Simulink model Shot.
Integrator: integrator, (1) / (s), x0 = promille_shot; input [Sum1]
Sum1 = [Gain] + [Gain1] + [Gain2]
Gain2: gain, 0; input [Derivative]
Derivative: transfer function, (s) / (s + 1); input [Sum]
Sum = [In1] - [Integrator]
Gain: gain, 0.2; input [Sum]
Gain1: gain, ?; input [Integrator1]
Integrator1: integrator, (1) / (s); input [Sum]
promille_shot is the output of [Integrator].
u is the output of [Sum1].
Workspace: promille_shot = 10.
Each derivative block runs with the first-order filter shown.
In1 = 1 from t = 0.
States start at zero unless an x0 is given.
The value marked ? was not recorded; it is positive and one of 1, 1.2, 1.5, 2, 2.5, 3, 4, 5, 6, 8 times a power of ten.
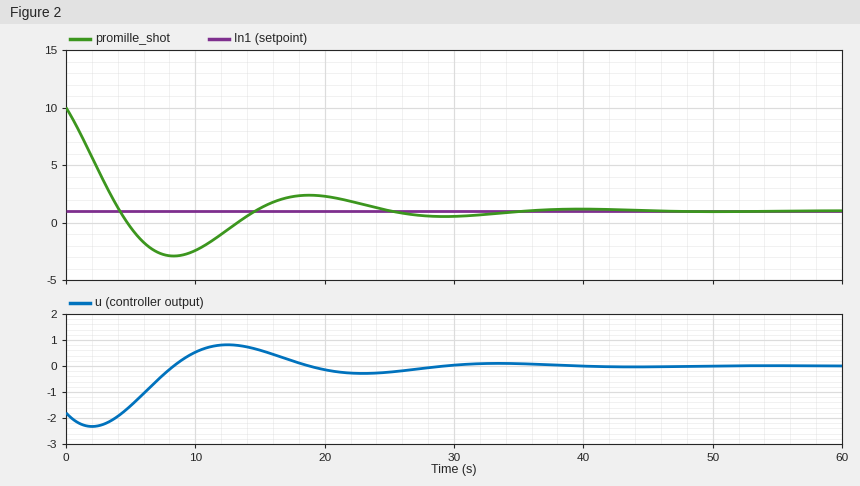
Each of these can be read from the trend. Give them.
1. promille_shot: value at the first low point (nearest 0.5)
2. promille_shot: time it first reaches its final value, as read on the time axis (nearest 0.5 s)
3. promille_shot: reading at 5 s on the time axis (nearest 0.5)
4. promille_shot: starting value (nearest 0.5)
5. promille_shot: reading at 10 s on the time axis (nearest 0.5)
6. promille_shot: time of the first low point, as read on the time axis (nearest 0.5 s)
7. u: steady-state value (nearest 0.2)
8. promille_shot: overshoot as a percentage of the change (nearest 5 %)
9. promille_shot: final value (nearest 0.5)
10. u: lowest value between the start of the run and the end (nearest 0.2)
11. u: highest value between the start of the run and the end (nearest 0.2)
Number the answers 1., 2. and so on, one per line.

1. -3.0
2. 4.0 s
3. -0.5
4. 10.0
5. -2.5
6. 8.5 s
7. 0.0
8. 45 %
9. 1.0
10. -2.4
11. 0.8
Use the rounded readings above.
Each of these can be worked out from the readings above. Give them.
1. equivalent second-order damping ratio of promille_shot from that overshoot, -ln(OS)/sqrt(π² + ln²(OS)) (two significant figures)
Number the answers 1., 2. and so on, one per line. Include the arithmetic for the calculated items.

1. ln(0.45) = -0.799; 0.799 / sqrt(9.870 + 0.638) = 0.25
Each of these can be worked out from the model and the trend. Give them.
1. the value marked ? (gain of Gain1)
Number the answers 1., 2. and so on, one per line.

1. 0.1
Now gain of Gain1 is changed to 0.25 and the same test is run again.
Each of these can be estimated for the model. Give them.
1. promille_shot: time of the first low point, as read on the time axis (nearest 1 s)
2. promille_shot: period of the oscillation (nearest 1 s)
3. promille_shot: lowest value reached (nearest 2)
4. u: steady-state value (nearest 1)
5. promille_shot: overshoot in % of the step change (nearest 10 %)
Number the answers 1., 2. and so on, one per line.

1. 6 s
2. 13 s
3. -4
4. 0
5. 60 %
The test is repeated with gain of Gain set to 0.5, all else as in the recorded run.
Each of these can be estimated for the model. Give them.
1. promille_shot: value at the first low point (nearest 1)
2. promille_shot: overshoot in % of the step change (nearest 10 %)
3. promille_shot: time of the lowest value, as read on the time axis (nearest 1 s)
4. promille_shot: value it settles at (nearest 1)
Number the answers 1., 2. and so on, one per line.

1. -1
2. 20 %
3. 7 s
4. 1
